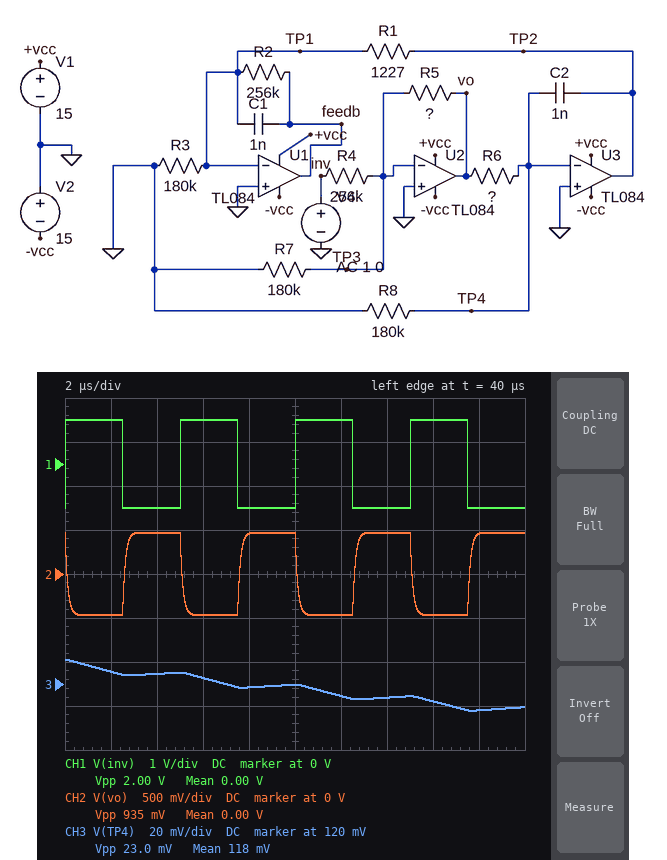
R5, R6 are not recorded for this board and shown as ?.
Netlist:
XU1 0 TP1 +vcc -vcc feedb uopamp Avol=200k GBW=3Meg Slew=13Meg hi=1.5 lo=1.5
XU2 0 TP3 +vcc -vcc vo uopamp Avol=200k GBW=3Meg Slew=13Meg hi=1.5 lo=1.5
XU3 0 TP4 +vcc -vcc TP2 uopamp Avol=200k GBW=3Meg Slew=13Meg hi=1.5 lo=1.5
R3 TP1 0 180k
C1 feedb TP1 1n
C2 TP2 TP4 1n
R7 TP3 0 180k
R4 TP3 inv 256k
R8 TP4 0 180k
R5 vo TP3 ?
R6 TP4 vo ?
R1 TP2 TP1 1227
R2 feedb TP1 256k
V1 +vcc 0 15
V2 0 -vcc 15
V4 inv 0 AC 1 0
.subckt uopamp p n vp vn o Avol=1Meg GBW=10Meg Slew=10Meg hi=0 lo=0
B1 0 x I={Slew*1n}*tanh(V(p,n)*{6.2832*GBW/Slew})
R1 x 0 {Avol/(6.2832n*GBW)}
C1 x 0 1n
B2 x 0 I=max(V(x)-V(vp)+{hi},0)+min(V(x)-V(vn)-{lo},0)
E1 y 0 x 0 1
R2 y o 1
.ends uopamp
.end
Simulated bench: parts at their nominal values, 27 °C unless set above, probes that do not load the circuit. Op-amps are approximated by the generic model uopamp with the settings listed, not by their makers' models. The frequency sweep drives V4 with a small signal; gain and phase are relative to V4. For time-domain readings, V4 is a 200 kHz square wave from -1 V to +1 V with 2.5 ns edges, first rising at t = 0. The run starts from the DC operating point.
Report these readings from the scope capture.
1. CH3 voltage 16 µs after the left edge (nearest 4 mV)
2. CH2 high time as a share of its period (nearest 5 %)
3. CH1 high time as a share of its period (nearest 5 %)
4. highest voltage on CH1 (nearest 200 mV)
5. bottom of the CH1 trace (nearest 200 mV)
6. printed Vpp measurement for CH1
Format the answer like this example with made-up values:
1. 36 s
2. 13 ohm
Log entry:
1. 112 mV
2. 50 %
3. 50 %
4. 1.0 V
5. -1.0 V
6. 2.00 V
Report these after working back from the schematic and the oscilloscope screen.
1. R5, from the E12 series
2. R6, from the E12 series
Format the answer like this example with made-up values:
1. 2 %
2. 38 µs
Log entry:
1. 120 kΩ
2. 270 kΩ
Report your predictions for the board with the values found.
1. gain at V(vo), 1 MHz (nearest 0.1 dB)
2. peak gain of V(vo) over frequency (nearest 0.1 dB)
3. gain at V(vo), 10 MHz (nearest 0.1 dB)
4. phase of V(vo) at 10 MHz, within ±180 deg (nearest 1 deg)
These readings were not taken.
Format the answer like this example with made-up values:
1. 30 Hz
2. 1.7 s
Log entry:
1. -8.4 dB
2. -6.6 dB
3. -23.7 dB
4. 98 deg
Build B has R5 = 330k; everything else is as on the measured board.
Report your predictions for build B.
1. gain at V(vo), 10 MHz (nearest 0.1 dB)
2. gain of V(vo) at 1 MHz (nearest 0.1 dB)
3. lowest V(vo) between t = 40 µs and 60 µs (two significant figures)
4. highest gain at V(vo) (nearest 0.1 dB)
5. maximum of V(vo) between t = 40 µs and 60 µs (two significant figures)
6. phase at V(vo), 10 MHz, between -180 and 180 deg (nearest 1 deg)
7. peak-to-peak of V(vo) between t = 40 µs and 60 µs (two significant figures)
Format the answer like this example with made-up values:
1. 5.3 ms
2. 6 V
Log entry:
1. -20.6 dB
2. -2.4 dB
3. -1.3 V
4. 2.2 dB
5. 1.3 V
6. 94 deg
7. 2.6 V
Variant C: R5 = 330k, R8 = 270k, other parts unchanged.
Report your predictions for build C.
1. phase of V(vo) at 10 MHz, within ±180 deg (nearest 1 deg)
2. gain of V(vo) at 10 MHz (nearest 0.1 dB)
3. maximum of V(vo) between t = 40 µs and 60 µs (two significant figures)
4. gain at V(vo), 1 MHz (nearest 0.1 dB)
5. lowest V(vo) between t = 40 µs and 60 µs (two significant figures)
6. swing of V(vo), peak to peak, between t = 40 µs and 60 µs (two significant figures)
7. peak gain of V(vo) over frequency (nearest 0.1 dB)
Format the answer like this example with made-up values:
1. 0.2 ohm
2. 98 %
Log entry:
1. 94 deg
2. -20.6 dB
3. 1.3 V
4. -2.4 dB
5. -1.3 V
6. 2.6 V
7. 2.2 dB
